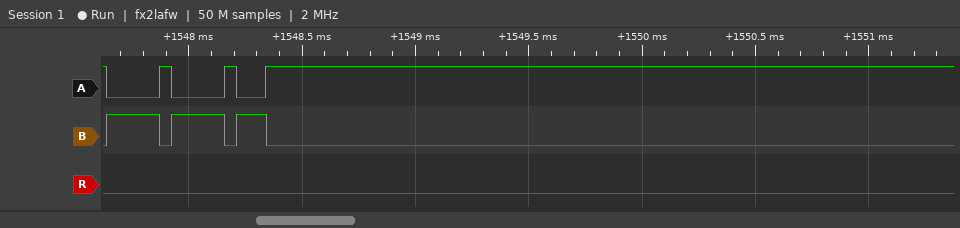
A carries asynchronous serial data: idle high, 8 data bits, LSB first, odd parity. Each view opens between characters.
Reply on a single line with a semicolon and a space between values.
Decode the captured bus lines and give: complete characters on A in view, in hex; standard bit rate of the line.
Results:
00, 00, F0; 38400 baud
